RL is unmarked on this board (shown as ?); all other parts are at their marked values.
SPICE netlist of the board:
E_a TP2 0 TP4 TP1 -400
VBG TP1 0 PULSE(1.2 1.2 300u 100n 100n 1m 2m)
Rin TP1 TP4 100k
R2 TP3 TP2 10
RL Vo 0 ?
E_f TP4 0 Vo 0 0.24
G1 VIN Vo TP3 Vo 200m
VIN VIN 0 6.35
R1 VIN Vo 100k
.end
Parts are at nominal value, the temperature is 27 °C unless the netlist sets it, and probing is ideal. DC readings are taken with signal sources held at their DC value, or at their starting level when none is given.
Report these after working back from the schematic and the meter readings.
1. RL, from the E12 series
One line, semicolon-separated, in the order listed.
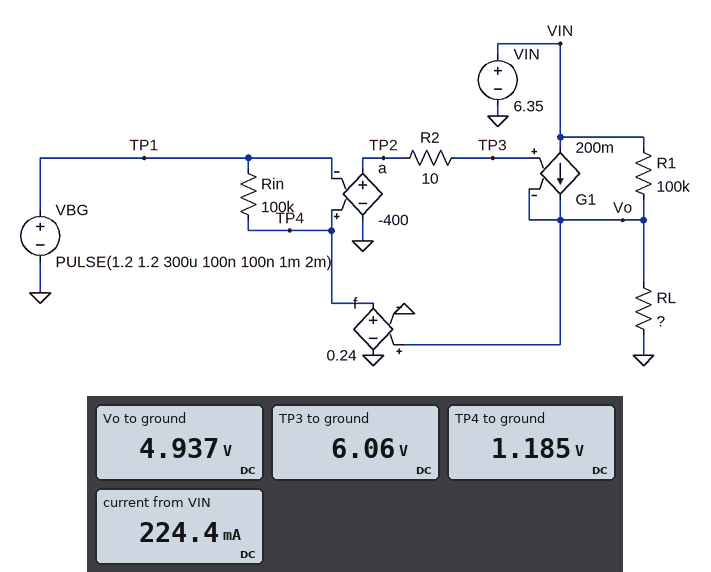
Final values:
22 Ω
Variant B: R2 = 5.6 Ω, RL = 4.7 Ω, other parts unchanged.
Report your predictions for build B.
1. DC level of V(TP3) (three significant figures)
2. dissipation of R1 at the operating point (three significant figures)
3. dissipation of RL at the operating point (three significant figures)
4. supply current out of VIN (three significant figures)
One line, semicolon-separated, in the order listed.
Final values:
10.1 V; 21.2 µW; 5.10 W; 1.04 A
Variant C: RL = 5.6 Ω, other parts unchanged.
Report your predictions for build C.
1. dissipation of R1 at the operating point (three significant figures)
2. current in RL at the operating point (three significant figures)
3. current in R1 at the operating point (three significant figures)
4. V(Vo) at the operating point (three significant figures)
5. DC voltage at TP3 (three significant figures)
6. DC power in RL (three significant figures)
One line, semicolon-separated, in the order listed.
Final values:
20.9 µW; 876 mA; 14.5 µA; 4.90 V; 9.28 V; 4.29 W
